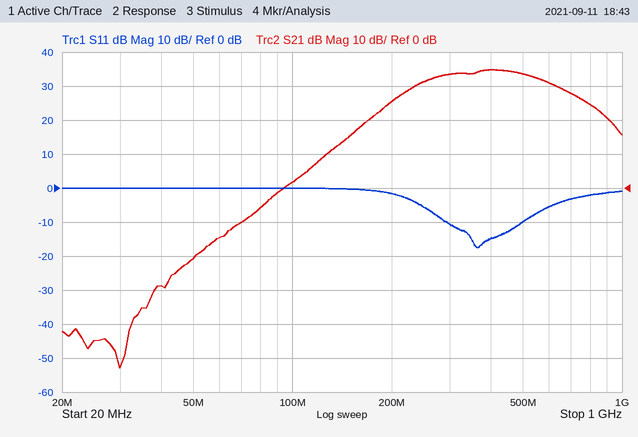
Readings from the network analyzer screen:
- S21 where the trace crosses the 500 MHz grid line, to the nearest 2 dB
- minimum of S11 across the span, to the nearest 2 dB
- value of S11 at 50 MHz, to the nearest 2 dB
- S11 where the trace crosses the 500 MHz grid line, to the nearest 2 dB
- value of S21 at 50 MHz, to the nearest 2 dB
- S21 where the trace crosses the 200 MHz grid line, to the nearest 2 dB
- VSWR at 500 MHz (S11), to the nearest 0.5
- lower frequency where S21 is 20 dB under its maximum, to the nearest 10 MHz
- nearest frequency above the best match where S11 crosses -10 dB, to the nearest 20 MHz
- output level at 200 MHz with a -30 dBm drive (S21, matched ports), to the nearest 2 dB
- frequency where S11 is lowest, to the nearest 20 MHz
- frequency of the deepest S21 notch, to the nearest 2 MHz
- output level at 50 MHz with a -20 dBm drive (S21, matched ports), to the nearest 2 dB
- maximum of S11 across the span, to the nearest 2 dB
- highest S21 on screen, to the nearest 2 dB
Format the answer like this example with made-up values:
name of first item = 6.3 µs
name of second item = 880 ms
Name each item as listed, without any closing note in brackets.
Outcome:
S21 where the trace crosses the 500 MHz grid line, to the nearest 2 dB = 34 dB
minimum of S11 across the span, to the nearest 2 dB = -18 dB
value of S11 at 50 MHz, to the nearest 2 dB = 0 dB
S11 where the trace crosses the 500 MHz grid line, to the nearest 2 dB = -10 dB
value of S21 at 50 MHz, to the nearest 2 dB = -20 dB
S21 where the trace crosses the 200 MHz grid line, to the nearest 2 dB = 26 dB
VSWR at 500 MHz (S11), to the nearest 0.5 = 2.0
lower frequency where S21 is 20 dB under its maximum, to the nearest 10 MHz = 150 MHz
nearest frequency above the best match where S11 crosses -10 dB, to the nearest 20 MHz = 500 MHz
output level at 200 MHz with a -30 dBm drive (S21, matched ports), to the nearest 2 dB = -4 dBm
frequency where S11 is lowest, to the nearest 20 MHz = 360 MHz
frequency of the deepest S21 notch, to the nearest 2 MHz = 30 MHz
output level at 50 MHz with a -20 dBm drive (S21, matched ports), to the nearest 2 dB = -40 dBm
maximum of S11 across the span, to the nearest 2 dB = 0 dB
highest S21 on screen, to the nearest 2 dB = 34 dB
